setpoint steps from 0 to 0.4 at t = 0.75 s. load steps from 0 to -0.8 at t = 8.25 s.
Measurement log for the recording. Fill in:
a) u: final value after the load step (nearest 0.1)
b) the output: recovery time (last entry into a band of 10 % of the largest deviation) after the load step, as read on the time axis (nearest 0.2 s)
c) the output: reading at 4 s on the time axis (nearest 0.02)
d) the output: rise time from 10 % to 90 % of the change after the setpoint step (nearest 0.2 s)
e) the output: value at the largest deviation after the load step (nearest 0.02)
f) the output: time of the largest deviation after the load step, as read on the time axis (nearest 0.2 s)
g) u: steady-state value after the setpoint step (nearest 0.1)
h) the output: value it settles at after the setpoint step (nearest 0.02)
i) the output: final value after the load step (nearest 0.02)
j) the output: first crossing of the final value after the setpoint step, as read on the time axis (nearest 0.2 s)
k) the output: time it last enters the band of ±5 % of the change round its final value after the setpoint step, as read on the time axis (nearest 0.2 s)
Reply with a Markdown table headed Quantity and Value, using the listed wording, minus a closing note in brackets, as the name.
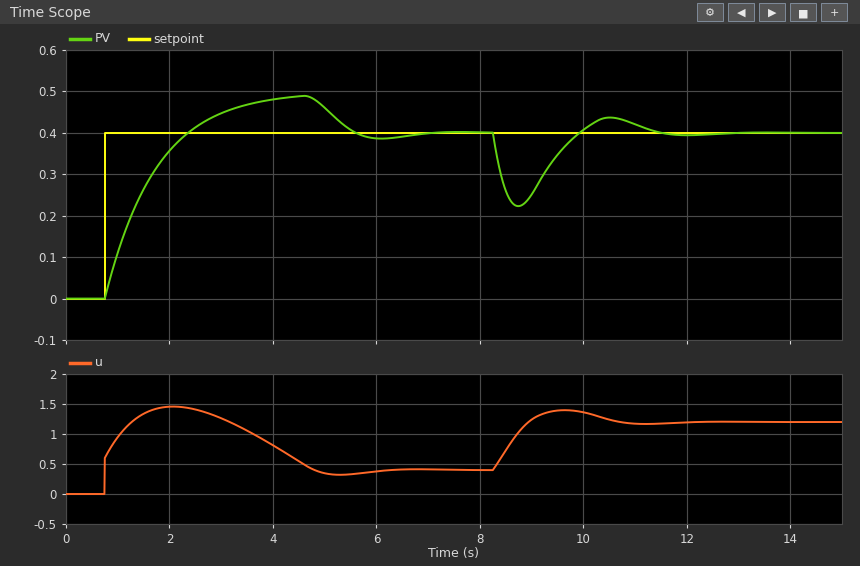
| Quantity | Value |
|---|---|
| u: final value after the load step | 1.2 |
| the output: recovery time (last entry into a band of 10 % of the largest deviation) after the load step, as read on the time axis | 11.0 s |
| the output: reading at 4 s on the time axis | 0.48 |
| the output: rise time from 10 % to 90 % of the change after the setpoint step | 1.2 s |
| the output: value at the largest deviation after the load step | 0.22 |
| the output: time of the largest deviation after the load step, as read on the time axis | 8.8 s |
| u: steady-state value after the setpoint step | 0.4 |
| the output: value it settles at after the setpoint step | 0.40 |
| the output: final value after the load step | 0.40 |
| the output: first crossing of the final value after the setpoint step, as read on the time axis | 2.4 s |
| the output: time it last enters the band of ±5 % of the change round its final value after the setpoint step, as read on the time axis | 5.4 s |
